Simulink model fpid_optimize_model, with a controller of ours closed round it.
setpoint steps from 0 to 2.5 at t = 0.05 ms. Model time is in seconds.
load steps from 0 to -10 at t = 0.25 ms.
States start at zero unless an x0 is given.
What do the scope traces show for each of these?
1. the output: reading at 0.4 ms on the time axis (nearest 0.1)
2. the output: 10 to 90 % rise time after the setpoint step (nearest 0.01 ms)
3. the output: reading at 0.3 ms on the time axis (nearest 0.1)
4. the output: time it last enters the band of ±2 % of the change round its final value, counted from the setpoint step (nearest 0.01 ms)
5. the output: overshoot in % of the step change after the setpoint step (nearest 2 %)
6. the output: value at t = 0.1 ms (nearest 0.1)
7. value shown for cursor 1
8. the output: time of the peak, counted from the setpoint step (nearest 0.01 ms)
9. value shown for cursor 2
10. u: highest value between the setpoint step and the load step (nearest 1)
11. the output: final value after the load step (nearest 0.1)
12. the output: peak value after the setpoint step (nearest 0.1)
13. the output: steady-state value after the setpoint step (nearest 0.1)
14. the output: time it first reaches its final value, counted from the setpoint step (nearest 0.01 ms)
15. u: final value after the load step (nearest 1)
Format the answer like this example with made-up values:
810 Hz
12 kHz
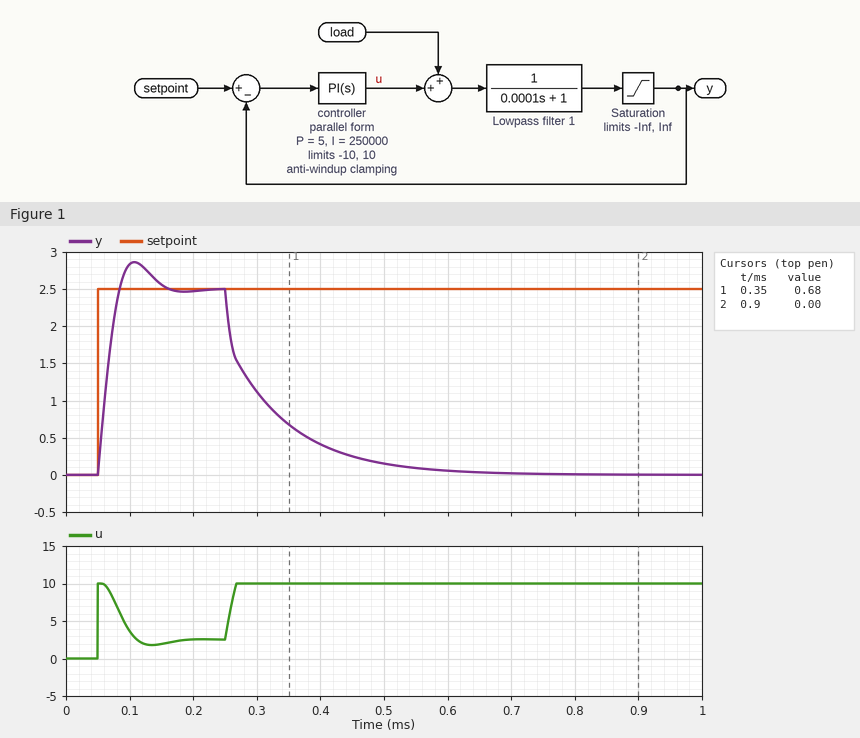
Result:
0.4
0.03 ms
1.1
0.10 ms
14 %
2.8
0.68
0.06 ms
0.00
10
0.0
2.9
2.5
0.03 ms
10
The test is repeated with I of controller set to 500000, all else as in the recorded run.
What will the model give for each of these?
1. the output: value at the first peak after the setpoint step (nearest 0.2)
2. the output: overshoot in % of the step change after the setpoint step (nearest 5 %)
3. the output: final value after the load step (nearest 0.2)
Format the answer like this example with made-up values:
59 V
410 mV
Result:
3.0
20 %
0.0
